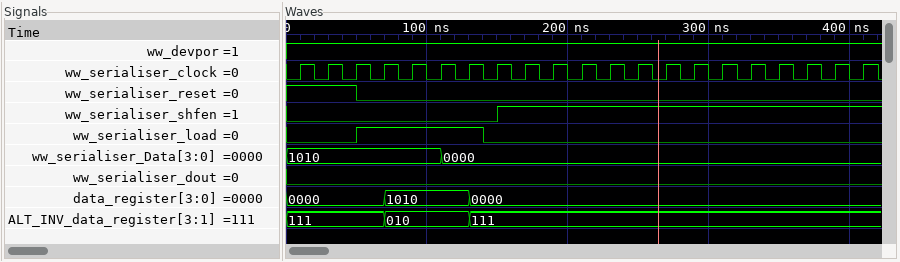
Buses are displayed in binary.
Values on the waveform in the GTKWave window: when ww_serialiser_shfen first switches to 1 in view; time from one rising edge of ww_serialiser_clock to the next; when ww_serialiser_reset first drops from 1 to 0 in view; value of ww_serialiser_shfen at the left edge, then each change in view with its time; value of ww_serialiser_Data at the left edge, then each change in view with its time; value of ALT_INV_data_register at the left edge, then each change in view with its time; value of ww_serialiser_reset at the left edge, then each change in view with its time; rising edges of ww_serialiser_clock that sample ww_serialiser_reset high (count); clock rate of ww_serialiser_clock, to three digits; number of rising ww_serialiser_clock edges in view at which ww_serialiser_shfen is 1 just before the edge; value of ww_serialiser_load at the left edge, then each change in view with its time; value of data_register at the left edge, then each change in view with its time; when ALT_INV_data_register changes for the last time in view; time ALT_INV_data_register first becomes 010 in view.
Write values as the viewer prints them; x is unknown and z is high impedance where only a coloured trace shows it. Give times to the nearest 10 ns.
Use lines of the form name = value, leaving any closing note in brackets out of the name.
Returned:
when ww_serialiser_shfen first switches to 1 in view = 150 ns
time from one rising edge of ww_serialiser_clock to the next = 20 ns
when ww_serialiser_reset first drops from 1 to 0 in view = 50 ns
value of ww_serialiser_shfen at the left edge, then each change in view with its time = 0, 1 at 150 ns
value of ww_serialiser_Data at the left edge, then each change in view with its time = 1010, 0000 at 110 ns
value of ALT_INV_data_register at the left edge, then each change in view with its time = 111, 010 at 70 ns, 111 at 130 ns
value of ww_serialiser_reset at the left edge, then each change in view with its time = 1, 0 at 50 ns
rising edges of ww_serialiser_clock that sample ww_serialiser_reset high = 3
clock rate of ww_serialiser_clock, to three digits = 50.0 MHz
number of rising ww_serialiser_clock edges in view at which ww_serialiser_shfen is 1 just before the edge = 13
value of ww_serialiser_load at the left edge, then each change in view with its time = 0, 1 at 50 ns, 0 at 140 ns
value of data_register at the left edge, then each change in view with its time = 0000, 1010 at 70 ns, 0000 at 130 ns
when ALT_INV_data_register changes for the last time in view = 130 ns
time ALT_INV_data_register first becomes 010 in view = 70 ns
